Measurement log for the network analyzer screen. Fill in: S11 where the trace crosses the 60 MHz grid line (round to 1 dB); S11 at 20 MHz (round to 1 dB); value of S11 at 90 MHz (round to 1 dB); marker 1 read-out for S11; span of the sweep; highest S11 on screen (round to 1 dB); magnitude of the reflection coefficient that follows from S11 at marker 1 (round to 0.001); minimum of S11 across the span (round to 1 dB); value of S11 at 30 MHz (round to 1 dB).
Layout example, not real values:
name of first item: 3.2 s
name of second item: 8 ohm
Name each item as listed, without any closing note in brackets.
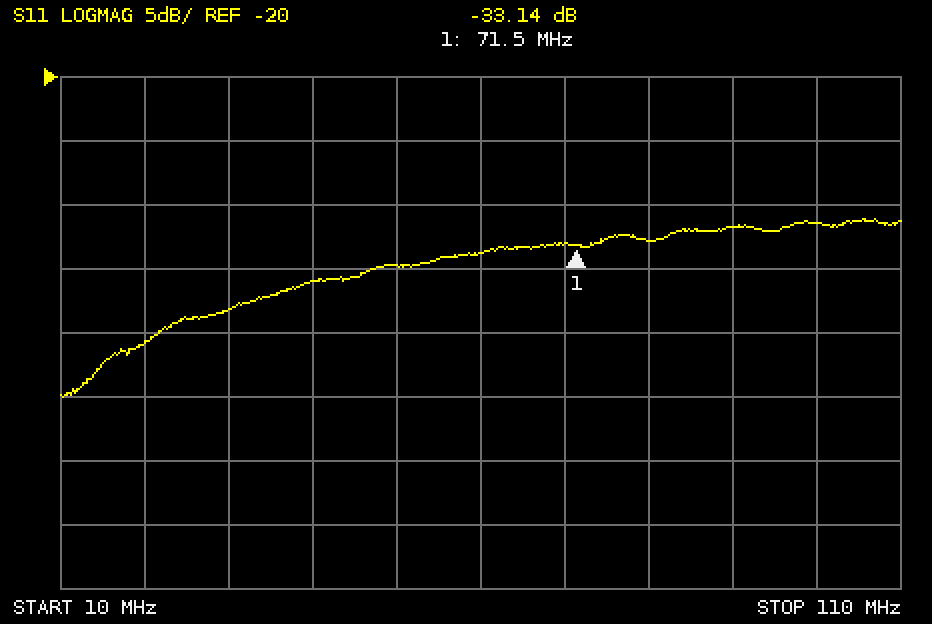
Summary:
S11 where the trace crosses the 60 MHz grid line: -34 dB
S11 at 20 MHz: -41 dB
value of S11 at 90 MHz: -32 dB
marker 1 read-out for S11: -33.14 dB
span of the sweep: 100 MHz
highest S11 on screen: -31 dB
magnitude of the reflection coefficient that follows from S11 at marker 1: 0.022
minimum of S11 across the span: -45 dB
value of S11 at 30 MHz: -38 dB
